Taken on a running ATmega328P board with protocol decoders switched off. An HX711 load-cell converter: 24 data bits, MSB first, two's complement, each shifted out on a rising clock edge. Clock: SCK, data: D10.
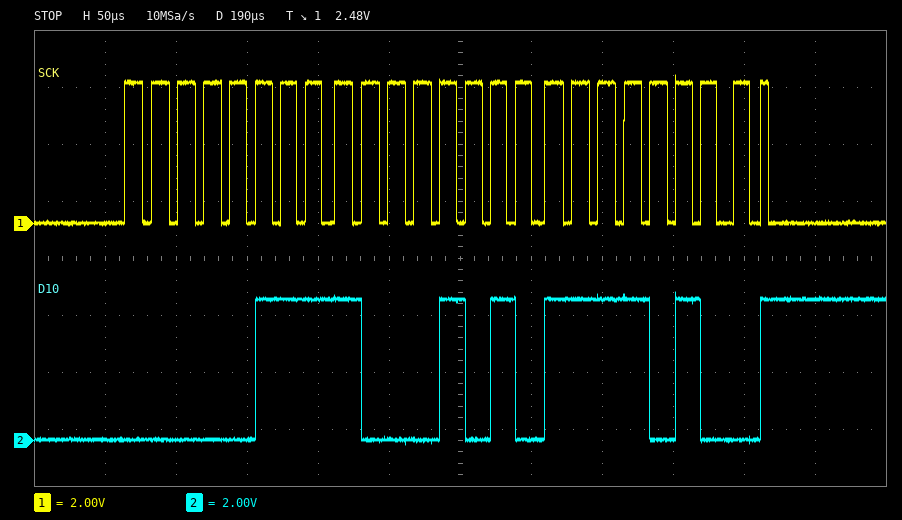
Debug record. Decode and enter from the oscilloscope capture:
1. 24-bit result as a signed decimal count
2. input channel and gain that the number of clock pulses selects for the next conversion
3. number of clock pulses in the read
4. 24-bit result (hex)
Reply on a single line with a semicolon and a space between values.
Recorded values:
494324; channel A, gain 128; 25; 0x078AF4
